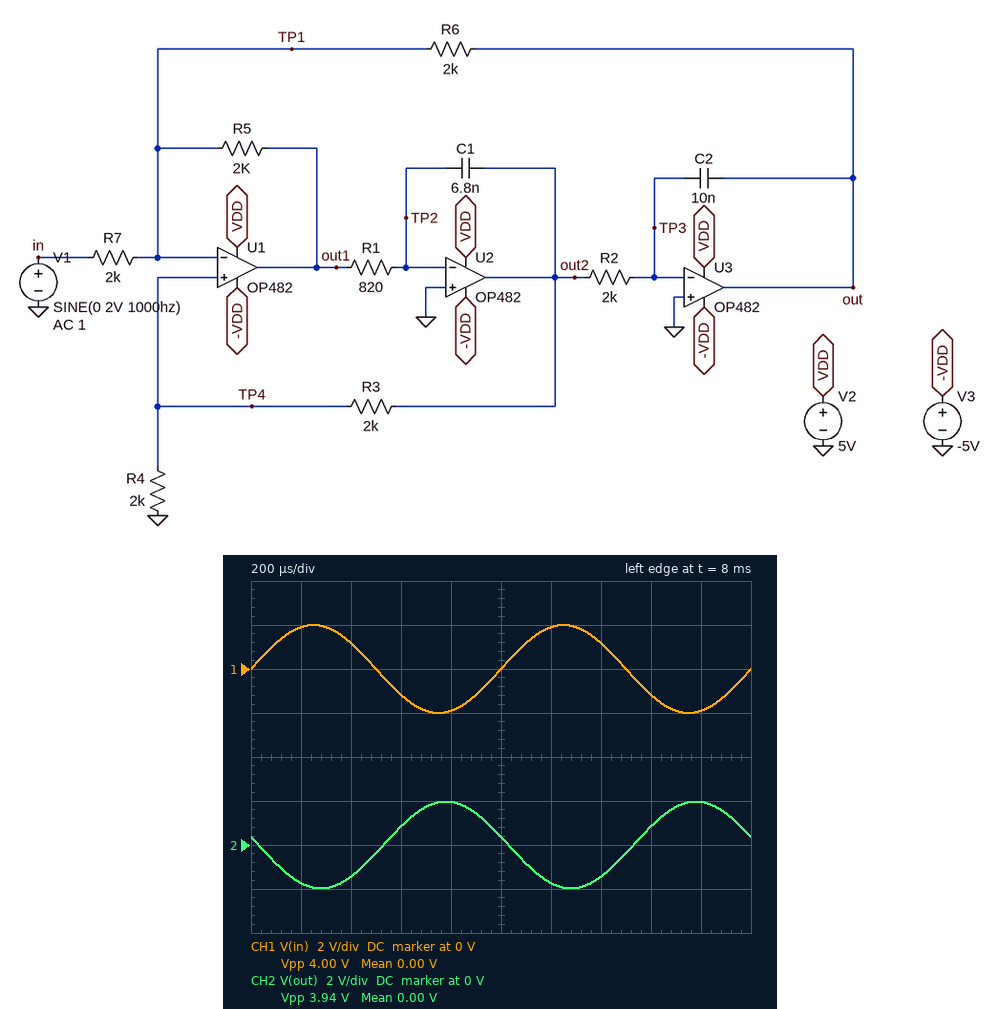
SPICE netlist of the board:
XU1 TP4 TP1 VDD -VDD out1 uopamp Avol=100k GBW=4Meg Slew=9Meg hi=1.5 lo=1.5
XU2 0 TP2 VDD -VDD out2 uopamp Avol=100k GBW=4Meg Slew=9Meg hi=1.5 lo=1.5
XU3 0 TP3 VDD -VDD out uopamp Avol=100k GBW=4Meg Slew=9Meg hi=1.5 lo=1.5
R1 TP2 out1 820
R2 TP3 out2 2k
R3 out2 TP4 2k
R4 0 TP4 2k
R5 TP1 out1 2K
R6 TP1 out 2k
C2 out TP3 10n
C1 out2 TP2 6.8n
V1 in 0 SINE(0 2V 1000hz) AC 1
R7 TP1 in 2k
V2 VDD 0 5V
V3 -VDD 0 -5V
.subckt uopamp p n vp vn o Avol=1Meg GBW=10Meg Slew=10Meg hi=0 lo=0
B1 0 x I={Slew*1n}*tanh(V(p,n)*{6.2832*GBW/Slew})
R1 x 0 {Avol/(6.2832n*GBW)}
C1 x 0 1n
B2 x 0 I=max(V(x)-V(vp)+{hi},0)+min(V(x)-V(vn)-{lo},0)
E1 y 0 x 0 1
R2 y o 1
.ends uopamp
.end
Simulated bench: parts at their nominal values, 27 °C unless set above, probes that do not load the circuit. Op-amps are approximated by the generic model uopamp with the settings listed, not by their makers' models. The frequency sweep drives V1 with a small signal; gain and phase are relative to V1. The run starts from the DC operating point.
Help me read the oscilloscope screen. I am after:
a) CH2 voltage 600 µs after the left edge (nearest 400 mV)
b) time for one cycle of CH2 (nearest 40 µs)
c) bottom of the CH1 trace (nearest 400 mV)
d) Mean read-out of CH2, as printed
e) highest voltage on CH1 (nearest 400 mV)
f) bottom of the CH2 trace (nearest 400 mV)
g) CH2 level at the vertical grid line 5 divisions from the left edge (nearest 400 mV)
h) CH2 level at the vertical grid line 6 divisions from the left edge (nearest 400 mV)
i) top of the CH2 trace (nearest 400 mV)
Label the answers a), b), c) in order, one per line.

a) 800 mV
b) 1.00 ms
c) -2.0 V
d) 0.00 V
e) 2.0 V
f) -2.0 V
g) 400 mV
h) -1.6 V
i) 2.0 V
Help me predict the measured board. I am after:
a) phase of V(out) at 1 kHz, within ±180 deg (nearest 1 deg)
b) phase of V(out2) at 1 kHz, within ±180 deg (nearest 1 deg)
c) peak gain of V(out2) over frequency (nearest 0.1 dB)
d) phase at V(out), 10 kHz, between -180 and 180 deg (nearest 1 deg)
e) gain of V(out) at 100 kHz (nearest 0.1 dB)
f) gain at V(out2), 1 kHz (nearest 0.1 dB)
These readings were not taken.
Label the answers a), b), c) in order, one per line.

a) 169 deg
b) 79 deg
c) -3.5 dB
d) 106 deg
e) -33.2 dB
f) -18.1 dB
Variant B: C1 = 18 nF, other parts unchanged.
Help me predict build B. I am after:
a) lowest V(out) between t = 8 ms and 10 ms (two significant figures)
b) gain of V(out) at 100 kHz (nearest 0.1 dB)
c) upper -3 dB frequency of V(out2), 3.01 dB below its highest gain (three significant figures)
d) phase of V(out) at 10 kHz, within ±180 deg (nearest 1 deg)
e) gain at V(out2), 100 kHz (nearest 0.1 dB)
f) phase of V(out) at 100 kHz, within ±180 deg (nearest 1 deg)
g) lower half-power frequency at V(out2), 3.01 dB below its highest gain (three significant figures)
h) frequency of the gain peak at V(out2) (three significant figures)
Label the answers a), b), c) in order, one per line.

a) -2.0 V
b) -41.3 dB
c) 20.5 kHz
d) 85 deg
e) -19.3 dB
f) 2 deg
g) 4.23 kHz
h) 9.32 kHz
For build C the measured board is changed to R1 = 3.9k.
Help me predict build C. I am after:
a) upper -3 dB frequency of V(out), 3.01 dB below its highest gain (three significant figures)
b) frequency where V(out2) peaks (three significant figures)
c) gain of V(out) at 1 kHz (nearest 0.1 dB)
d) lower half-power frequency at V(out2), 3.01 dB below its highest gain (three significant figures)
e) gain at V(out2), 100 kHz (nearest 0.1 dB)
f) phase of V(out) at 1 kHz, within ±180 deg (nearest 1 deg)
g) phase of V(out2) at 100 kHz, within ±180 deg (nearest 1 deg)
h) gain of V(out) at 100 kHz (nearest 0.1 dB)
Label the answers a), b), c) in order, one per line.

a) 7.41 kHz
b) 6.93 kHz
c) 0 dB
d) 3.76 kHz
e) -24.4 dB
f) 169 deg
g) -91 deg
h) -46.4 dB
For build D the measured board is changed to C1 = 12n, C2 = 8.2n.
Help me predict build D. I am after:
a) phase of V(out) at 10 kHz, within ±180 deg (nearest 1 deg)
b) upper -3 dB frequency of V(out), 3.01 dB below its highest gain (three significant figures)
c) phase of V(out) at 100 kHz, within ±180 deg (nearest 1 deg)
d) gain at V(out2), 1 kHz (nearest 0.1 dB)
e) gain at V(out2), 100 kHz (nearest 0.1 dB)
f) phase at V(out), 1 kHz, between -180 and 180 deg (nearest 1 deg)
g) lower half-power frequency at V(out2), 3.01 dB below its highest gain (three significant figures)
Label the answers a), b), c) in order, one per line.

a) 103 deg
b) 8.48 kHz
c) 7 deg
d) -19.8 dB
e) -15.8 dB
f) 171 deg
g) 5.34 kHz
